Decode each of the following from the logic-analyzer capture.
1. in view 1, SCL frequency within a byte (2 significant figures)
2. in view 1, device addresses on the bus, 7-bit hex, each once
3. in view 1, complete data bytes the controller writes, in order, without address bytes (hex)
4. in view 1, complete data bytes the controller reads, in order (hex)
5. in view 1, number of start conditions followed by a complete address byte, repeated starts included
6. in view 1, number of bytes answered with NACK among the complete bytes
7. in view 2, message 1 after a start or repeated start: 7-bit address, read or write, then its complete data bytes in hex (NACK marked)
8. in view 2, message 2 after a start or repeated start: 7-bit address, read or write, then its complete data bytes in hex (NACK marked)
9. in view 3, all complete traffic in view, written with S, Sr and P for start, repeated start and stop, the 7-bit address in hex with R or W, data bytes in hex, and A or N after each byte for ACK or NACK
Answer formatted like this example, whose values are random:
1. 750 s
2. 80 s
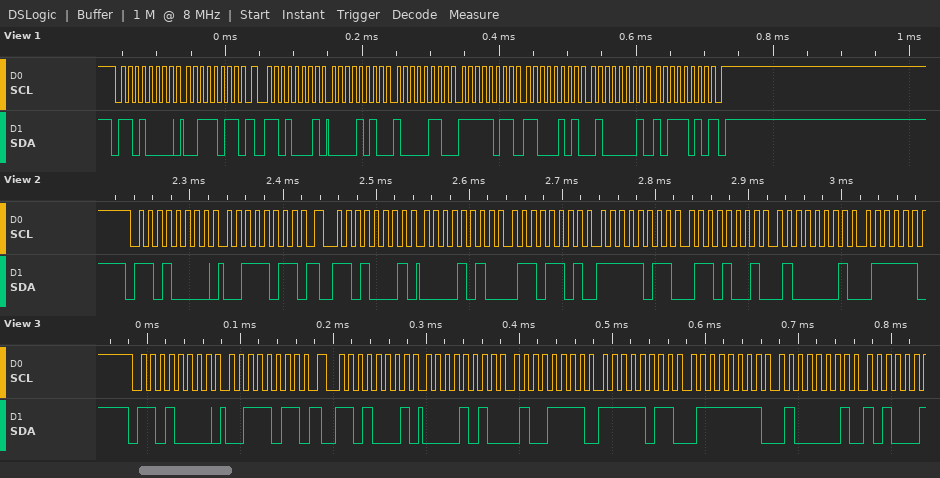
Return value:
1. 100 kHz
2. 0x68
3. 3B
4. 0A 86 FB C5 41 BA
5. 2
6. 1
7. 0x68 write: 3B
8. 0x68 read: 0A 6D FB 69 41
9. S 68W A 3B A Sr 68R A 0A A 4F A FB A 7F A 41 A
